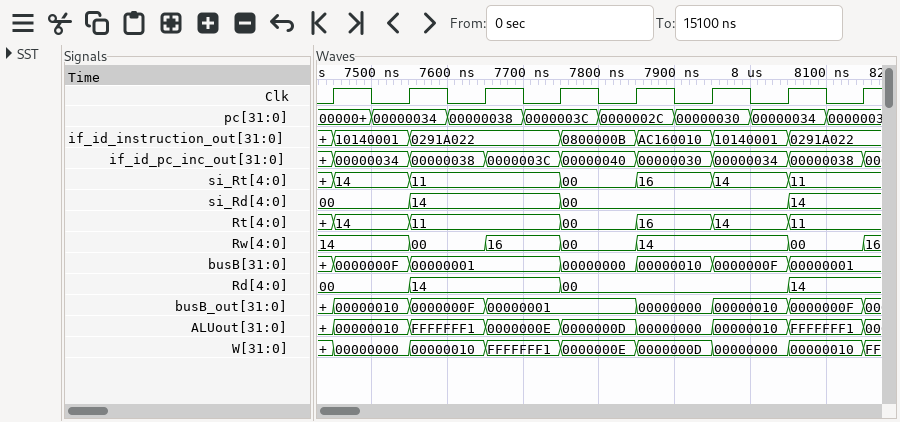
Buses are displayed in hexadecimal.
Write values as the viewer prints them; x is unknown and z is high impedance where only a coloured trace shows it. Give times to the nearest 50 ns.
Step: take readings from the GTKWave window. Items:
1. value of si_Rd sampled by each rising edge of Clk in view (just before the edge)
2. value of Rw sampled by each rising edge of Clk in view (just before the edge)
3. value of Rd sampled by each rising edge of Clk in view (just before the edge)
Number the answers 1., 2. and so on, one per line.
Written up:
1. 00, 00, 14, 14, 00, 00, 00, 14
2. 14, 14, 00, 16, 00, 14, 14, 00
3. 00, 00, 14, 14, 00, 00, 00, 14
